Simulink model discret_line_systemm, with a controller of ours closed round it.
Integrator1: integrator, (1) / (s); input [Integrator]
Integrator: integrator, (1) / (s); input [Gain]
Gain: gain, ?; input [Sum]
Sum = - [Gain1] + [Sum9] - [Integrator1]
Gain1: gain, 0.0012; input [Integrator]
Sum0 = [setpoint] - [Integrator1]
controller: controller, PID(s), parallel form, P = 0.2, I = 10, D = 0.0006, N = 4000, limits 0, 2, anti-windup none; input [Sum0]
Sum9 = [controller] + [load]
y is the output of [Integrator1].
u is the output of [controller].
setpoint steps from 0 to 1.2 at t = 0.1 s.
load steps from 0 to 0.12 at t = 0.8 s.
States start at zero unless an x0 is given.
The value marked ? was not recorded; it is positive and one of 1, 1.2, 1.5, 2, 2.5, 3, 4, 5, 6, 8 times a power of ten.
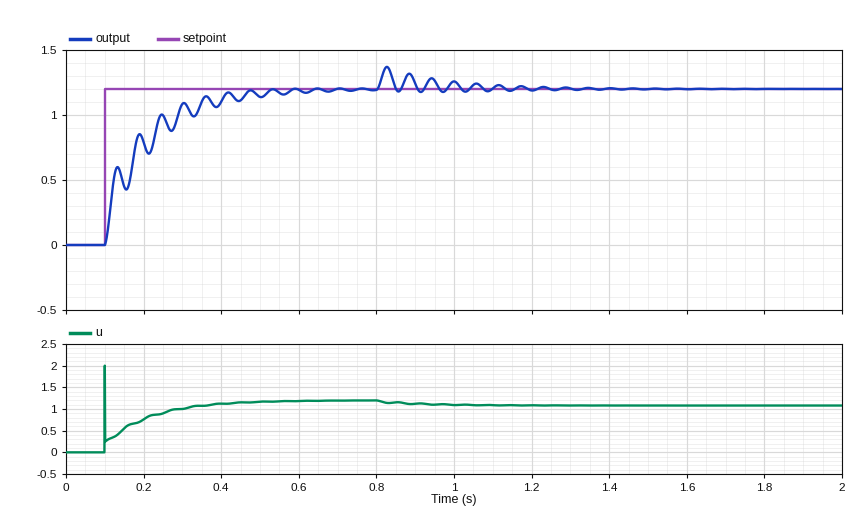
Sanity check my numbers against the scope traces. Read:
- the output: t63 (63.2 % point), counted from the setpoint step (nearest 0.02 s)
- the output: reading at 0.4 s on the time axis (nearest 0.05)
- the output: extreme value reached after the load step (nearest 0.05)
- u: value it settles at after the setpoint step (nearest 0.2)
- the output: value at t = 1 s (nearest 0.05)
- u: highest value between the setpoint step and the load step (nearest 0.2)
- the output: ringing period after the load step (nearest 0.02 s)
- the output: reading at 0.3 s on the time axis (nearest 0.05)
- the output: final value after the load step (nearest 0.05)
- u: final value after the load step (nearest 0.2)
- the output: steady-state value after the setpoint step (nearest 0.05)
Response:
0.08 s
1.10
1.35
1.2
1.25
2.0
0.06 s
1.10
1.20
1.0
1.20
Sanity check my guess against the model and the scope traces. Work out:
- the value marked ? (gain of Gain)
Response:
10000
